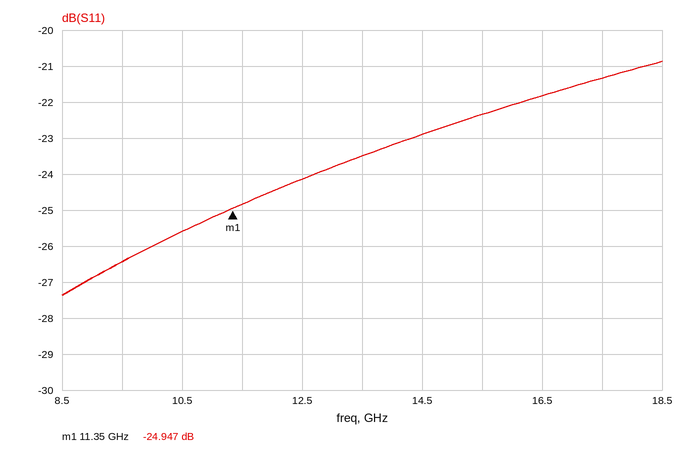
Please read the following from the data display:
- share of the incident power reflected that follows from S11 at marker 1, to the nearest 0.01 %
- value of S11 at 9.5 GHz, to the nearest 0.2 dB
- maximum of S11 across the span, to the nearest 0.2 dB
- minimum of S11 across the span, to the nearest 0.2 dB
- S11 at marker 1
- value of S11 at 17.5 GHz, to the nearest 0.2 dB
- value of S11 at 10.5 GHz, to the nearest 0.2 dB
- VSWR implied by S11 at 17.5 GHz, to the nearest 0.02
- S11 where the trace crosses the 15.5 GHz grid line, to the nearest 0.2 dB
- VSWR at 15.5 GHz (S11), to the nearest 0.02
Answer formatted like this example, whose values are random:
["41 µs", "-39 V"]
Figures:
["0.32 %", "-26.4 dB", "-20.8 dB", "-27.4 dB", "-24.947 dB", "-21.4 dB", "-25.6 dB", "1.18", "-22.4 dB", "1.16"]
